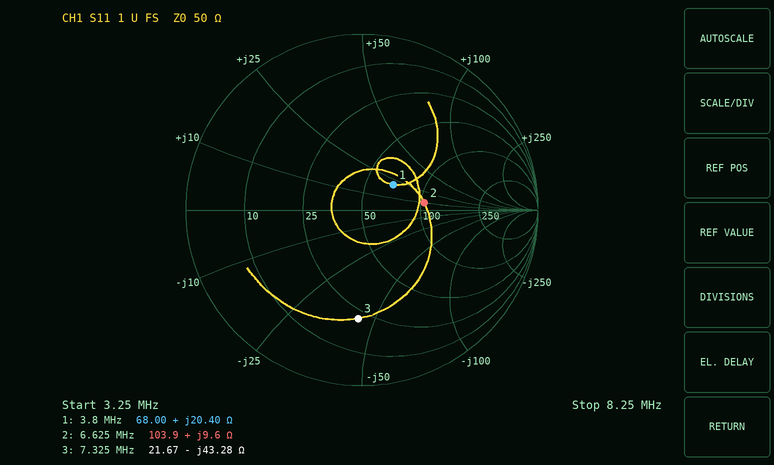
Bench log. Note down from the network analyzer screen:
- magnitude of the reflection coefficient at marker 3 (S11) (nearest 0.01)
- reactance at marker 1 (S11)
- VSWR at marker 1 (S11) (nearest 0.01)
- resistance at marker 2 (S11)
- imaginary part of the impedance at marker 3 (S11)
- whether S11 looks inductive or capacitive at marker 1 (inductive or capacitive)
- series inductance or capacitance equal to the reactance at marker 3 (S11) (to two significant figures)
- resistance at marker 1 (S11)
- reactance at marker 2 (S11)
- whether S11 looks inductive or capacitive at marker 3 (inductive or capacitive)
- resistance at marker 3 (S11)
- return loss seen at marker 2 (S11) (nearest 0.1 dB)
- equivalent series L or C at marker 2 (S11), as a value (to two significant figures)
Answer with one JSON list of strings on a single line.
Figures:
["0.62", "+20.40 Ω", "1.59", "103.9 Ω", "-43.28 Ω", "inductive", "500 pF", "68.00 Ω", "+9.6 Ω", "capacitive", "21.67 Ω", "9.0 dB", "230 nH"]
